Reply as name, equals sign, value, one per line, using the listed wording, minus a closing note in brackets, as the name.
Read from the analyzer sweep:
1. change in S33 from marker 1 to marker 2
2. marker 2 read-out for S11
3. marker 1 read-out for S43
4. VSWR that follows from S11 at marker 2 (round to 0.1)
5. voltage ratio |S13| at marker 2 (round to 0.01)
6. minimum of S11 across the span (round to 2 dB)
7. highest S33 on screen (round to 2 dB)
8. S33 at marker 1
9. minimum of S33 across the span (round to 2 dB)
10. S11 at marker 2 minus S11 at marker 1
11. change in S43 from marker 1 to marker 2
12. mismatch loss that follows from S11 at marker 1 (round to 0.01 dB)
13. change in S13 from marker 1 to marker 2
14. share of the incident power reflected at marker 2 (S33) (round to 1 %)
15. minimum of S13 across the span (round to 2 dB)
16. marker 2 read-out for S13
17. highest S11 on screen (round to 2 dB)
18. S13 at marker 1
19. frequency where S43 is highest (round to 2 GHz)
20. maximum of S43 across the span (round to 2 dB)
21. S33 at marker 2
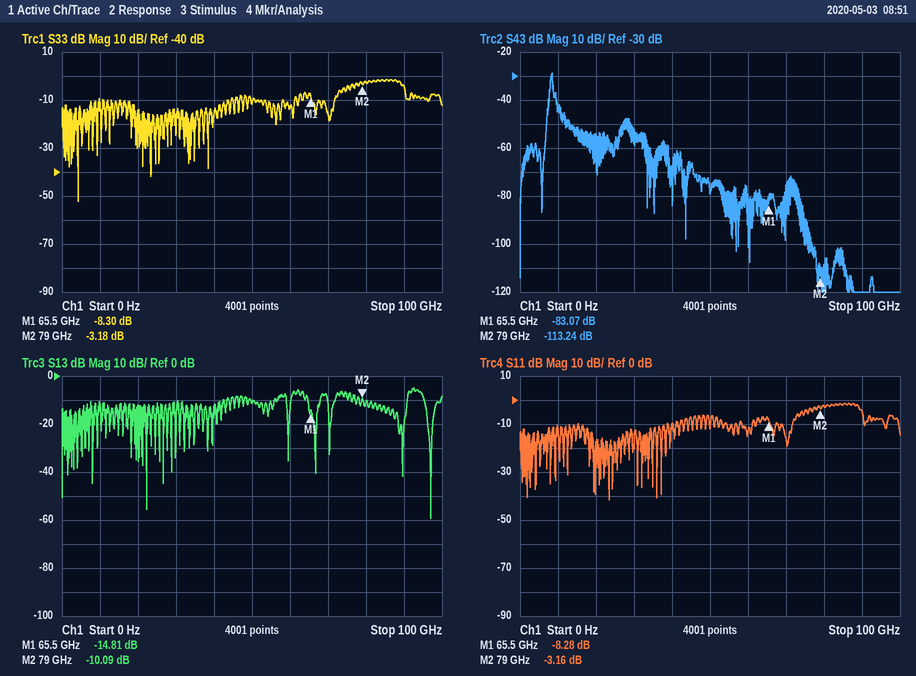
change in S33 from marker 1 to marker 2 = 5.12 dB
marker 2 read-out for S11 = -3.16 dB
marker 1 read-out for S43 = -83.07 dB
VSWR that follows from S11 at marker 2 = 5.6
voltage ratio |S13| at marker 2 = 0.31
minimum of S11 across the span = -42 dB
highest S33 on screen = -2 dB
S33 at marker 1 = -8.30 dB
minimum of S33 across the span = -52 dB
S11 at marker 2 minus S11 at marker 1 = 5.12 dB
change in S43 from marker 1 to marker 2 = -30.17 dB
mismatch loss that follows from S11 at marker 1 = 0.70 dB
change in S13 from marker 1 to marker 2 = 4.72 dB
share of the incident power reflected at marker 2 (S33) = 48 %
minimum of S13 across the span = -60 dB
marker 2 read-out for S13 = -10.09 dB
highest S11 on screen = -2 dB
S13 at marker 1 = -14.81 dB
frequency where S43 is highest = 8 GHz
maximum of S43 across the span = -28 dB
S33 at marker 2 = -3.18 dB
